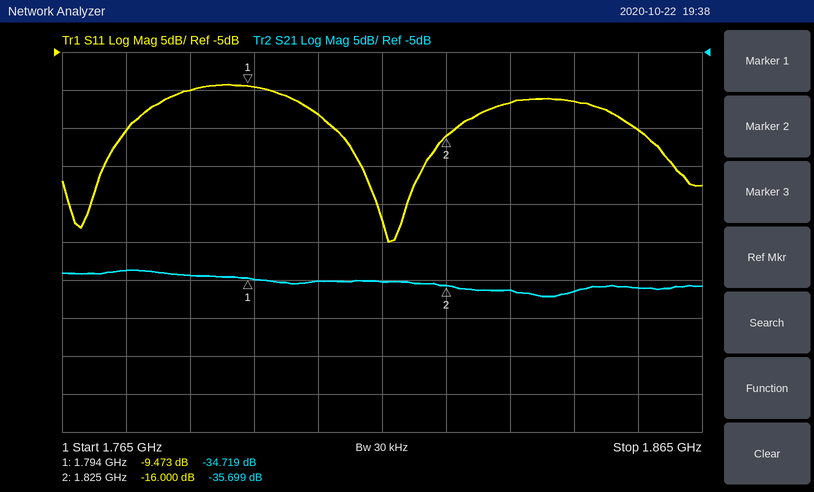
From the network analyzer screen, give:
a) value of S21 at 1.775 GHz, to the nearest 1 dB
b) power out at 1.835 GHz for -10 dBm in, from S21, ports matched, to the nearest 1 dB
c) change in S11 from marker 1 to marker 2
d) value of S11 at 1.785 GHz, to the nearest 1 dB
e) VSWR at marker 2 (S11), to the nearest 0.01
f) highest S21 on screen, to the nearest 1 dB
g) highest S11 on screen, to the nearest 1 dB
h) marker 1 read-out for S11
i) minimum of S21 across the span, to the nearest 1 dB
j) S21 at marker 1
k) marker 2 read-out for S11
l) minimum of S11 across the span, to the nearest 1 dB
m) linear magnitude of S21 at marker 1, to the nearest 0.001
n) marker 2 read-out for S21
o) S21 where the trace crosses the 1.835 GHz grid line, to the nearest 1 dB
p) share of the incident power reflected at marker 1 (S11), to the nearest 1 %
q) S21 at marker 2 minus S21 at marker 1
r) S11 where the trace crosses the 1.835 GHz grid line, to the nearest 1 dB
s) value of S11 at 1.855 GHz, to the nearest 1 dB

-34 dB
-46 dBm
-6.527 dB
-10 dB
1.38
-34 dB
-9 dB
-9.473 dB
-37 dB
-34.719 dB
-16.000 dB
-30 dB
0.018
-35.699 dB
-36 dB
11 %
-0.980 dB
-12 dB
-15 dB
